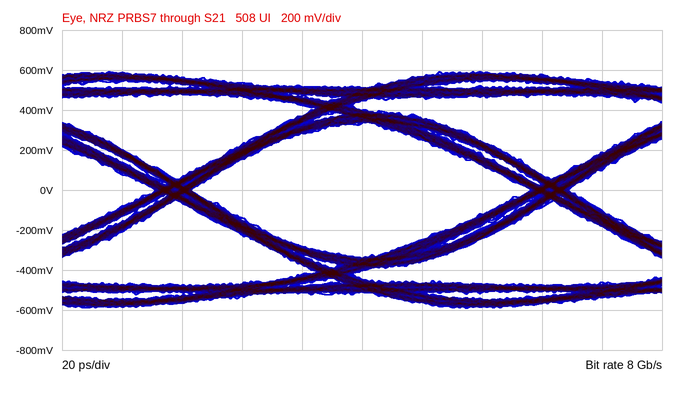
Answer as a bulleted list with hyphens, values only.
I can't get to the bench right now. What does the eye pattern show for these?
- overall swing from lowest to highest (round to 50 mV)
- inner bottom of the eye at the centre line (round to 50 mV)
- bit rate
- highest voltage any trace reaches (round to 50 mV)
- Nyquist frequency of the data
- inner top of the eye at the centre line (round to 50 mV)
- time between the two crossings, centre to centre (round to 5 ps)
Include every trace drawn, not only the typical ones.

- 1.20 V
- -350 mV
- 8 Gb/s
- 600 mV
- 4 GHz
- 350 mV
- 125 ps
